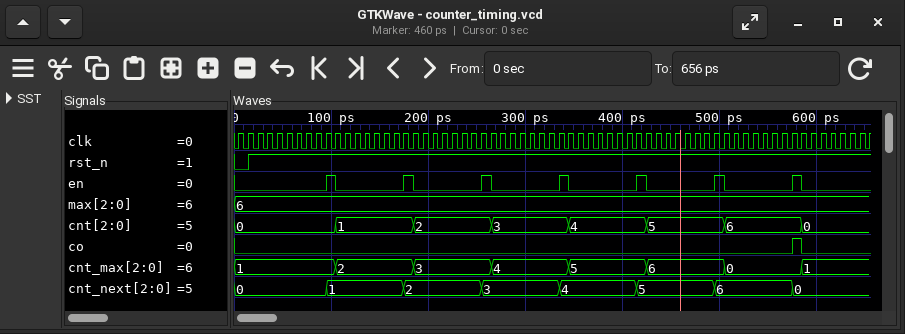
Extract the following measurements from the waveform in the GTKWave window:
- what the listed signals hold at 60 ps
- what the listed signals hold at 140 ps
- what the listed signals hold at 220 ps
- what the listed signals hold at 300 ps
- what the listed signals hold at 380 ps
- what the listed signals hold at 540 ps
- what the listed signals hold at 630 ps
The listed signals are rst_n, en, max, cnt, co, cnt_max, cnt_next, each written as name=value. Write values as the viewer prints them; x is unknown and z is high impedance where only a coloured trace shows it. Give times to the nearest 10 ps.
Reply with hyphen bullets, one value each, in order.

- rst_n=1, en=0, max=6, cnt=0, co=0, cnt_max=1, cnt_next=0
- rst_n=1, en=0, max=6, cnt=1, co=0, cnt_max=2, cnt_next=1
- rst_n=1, en=0, max=6, cnt=2, co=0, cnt_max=3, cnt_next=2
- rst_n=1, en=0, max=6, cnt=3, co=0, cnt_max=4, cnt_next=3
- rst_n=1, en=0, max=6, cnt=4, co=0, cnt_max=5, cnt_next=4
- rst_n=1, en=0, max=6, cnt=6, co=0, cnt_max=0, cnt_next=6
- rst_n=1, en=0, max=6, cnt=0, co=0, cnt_max=1, cnt_next=0
